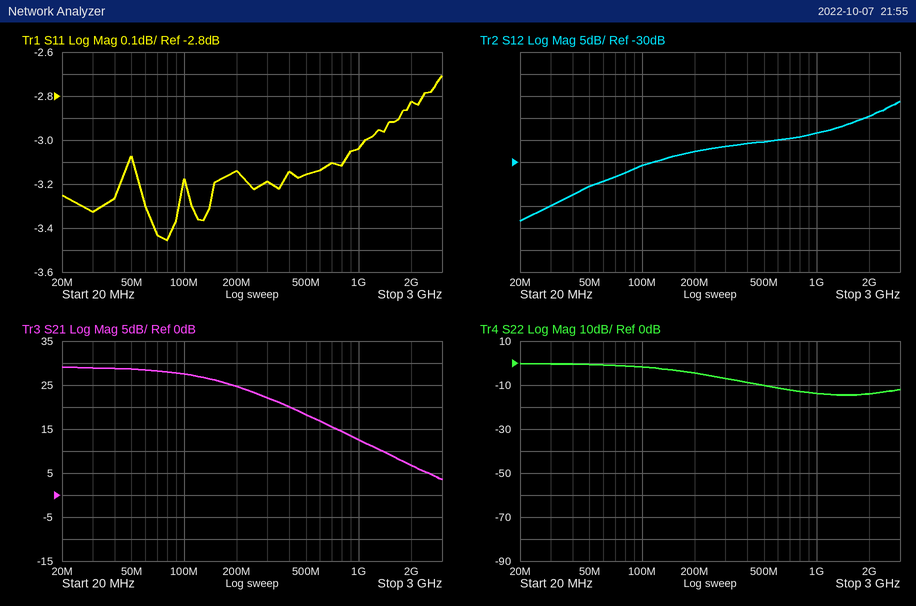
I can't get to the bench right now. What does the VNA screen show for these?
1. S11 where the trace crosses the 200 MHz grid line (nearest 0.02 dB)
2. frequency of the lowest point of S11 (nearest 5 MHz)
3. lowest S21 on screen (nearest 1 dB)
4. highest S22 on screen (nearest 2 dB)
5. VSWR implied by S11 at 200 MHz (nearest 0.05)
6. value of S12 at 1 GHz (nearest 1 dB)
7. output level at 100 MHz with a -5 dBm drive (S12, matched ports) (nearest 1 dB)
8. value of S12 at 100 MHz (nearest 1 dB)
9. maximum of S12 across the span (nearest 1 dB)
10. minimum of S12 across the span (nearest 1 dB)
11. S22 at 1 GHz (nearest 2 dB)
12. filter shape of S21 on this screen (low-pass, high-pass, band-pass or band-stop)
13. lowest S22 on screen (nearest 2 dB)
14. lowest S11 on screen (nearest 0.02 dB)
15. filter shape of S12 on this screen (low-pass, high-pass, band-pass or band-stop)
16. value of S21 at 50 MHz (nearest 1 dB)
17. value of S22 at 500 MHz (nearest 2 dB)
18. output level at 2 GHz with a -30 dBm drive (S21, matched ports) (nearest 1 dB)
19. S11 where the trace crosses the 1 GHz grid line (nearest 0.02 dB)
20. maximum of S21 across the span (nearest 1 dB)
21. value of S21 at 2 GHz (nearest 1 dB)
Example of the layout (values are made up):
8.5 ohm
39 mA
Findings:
-3.14 dB
80 MHz
4 dB
0 dB
5.60
-23 dB
-36 dBm
-31 dB
-16 dB
-43 dB
-14 dB
low-pass
-14 dB
-3.46 dB
high-pass
29 dB
-10 dB
-23 dBm
-3.04 dB
29 dB
7 dB
